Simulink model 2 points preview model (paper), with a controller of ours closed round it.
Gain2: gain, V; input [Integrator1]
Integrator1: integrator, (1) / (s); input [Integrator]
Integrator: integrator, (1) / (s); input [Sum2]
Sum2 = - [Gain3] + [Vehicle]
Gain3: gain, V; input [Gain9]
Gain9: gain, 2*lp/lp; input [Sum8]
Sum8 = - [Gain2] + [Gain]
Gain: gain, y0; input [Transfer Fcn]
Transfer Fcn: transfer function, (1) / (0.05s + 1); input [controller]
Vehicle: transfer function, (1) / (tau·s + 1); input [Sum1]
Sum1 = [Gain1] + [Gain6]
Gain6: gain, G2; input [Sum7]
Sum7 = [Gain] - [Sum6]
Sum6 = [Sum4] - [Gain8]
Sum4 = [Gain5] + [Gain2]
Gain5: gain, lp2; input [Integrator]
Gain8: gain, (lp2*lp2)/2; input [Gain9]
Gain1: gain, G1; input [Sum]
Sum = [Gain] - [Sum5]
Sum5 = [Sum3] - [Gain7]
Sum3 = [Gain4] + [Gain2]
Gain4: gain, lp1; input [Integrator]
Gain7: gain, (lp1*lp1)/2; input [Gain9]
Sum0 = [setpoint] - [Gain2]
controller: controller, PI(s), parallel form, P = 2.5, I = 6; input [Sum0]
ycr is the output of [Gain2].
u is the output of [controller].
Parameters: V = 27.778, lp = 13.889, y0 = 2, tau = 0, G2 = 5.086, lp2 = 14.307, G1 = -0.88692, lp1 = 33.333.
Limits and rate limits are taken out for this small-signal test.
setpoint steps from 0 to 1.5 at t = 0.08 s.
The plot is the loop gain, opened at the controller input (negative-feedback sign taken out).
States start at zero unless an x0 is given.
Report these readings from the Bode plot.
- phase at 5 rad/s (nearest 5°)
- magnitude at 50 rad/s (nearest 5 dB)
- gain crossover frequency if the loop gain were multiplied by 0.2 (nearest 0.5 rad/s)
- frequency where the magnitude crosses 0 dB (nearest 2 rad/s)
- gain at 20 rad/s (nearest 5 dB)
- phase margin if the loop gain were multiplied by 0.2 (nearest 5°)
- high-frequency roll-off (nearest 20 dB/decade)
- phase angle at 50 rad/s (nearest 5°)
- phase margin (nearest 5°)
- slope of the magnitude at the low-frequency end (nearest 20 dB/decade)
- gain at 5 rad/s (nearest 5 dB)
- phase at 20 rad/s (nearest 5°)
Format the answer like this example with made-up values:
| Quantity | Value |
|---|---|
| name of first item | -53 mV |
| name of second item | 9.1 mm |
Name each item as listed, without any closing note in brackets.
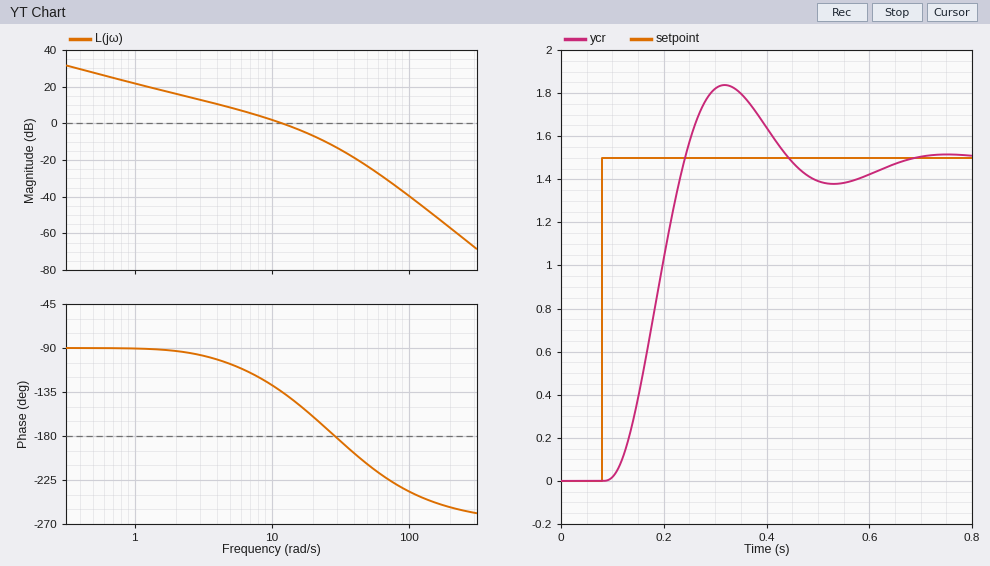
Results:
| Quantity | Value |
|---|---|
| phase at 5 rad/s | -105° |
| magnitude at 50 rad/s | -25 dB |
| gain crossover frequency if the loop gain were multiplied by 0.2 | 2.5 rad/s |
| frequency where the magnitude crosses 0 dB | 12 rad/s |
| gain at 20 rad/s | -5 dB |
| phase margin if the loop gain were multiplied by 0.2 | 85° |
| high-frequency roll-off | -60 dB/decade |
| phase angle at 50 rad/s | -210° |
| phase margin | 45° |
| slope of the magnitude at the low-frequency end | -20 dB/decade |
| gain at 5 rad/s | 10 dB |
| phase at 20 rad/s | -160° |
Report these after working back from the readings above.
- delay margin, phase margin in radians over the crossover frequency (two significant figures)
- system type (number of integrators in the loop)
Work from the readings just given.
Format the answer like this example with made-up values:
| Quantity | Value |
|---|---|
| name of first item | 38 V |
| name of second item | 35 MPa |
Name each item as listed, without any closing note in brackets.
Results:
| Quantity | Value |
|---|---|
| delay margin, phase margin in radians over the crossover frequency | 0.065 s |
| system type | 1 |
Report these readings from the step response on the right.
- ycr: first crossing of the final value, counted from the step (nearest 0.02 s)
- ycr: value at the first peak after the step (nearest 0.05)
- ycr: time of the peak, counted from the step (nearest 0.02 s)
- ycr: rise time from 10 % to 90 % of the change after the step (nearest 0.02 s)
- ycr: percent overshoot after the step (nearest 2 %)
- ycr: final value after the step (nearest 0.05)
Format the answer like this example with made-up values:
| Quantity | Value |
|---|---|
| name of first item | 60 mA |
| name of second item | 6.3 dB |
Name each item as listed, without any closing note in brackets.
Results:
| Quantity | Value |
|---|---|
| ycr: first crossing of the final value, counted from the step | 0.16 s |
| ycr: value at the first peak after the step | 1.85 |
| ycr: time of the peak, counted from the step | 0.24 s |
| ycr: rise time from 10 % to 90 % of the change after the step | 0.10 s |
| ycr: percent overshoot after the step | 22 % |
| ycr: final value after the step | 1.50 |
